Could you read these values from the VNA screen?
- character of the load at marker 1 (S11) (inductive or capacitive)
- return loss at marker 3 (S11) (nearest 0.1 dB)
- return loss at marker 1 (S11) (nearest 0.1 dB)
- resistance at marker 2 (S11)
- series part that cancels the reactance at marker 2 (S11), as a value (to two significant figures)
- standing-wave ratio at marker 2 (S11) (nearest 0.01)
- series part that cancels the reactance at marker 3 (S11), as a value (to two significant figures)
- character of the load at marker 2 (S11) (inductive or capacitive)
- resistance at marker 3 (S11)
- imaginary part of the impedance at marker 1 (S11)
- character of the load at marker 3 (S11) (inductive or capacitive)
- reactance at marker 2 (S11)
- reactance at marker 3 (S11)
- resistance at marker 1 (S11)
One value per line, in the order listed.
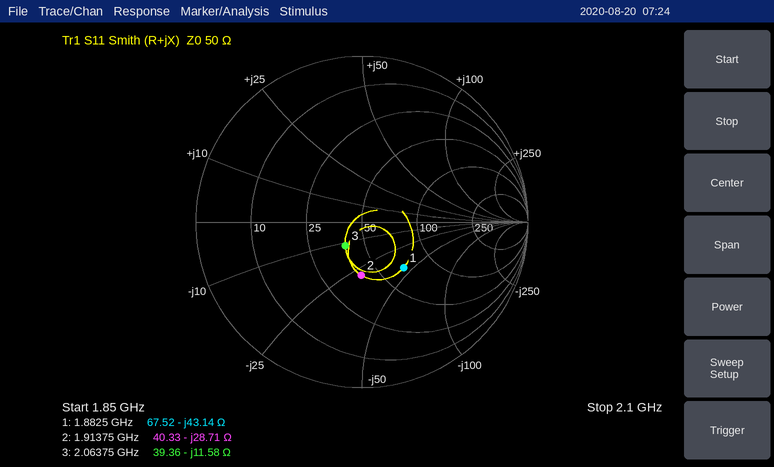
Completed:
capacitive
15.2 dB
8.6 dB
40.33 Ω
2.4 nH
1.94
890 pH
capacitive
39.36 Ω
-43.14 Ω
capacitive
-28.71 Ω
-11.58 Ω
67.52 Ω
